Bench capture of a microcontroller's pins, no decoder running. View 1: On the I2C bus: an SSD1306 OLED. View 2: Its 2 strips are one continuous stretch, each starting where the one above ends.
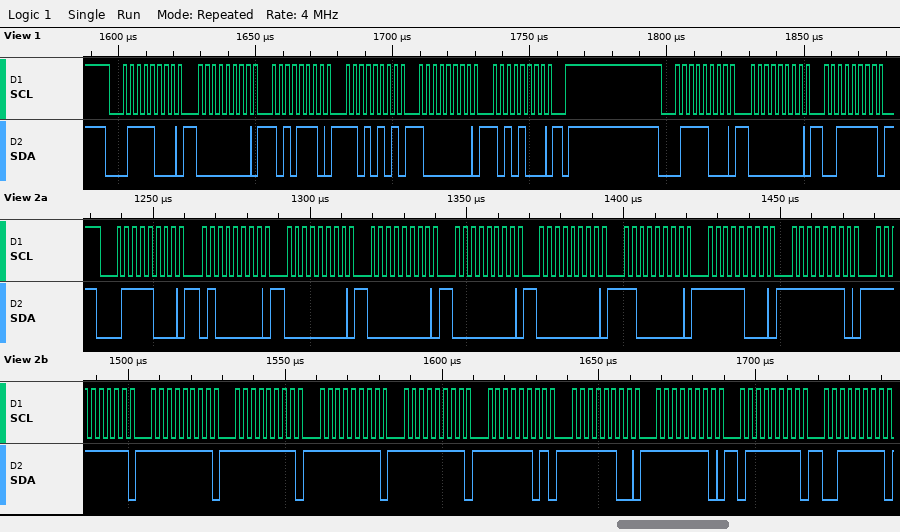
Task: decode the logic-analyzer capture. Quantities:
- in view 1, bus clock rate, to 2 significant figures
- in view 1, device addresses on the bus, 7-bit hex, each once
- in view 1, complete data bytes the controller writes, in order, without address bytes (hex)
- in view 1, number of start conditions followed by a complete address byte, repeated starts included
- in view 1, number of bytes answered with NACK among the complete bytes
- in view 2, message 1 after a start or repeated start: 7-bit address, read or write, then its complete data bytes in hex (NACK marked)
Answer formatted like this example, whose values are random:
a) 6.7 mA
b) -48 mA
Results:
a) 400 kHz
b) 0x3C
c) 00 AE D5 80 A8 00 3F
d) 2
e) 0
f) 0x3C write: 40 00 00 00 00 C0 F8 FE FF FF FF FF FF FD FC FE 7F 3F
